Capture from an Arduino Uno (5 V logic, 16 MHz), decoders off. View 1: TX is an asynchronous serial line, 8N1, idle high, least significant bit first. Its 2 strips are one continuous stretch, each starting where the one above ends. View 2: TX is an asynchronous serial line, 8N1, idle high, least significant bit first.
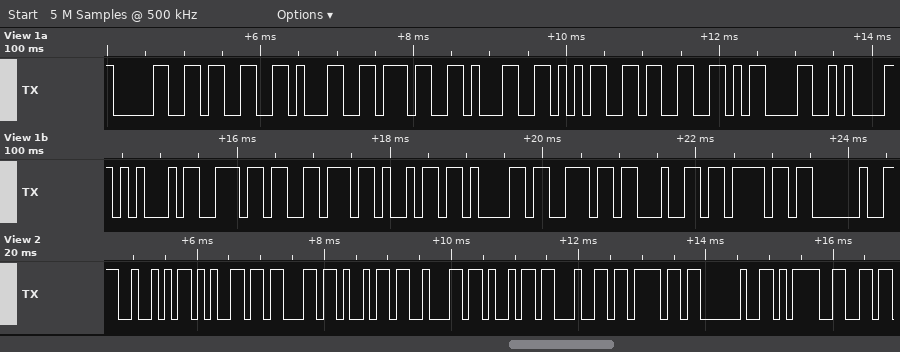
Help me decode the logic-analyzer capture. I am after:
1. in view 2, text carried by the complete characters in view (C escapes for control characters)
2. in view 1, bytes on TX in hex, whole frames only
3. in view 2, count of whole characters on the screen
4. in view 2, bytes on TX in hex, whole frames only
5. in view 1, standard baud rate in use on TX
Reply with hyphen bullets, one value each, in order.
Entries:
- "Recibido ="
- 0x30 0x33 0x31 0x37 0x31 0x35 0x33 0x0D 0x0A 0x45 0x6E 0x76 0x69 0x61 0x6E 0x64 0x6F 0x20
- 10
- 52 65 63 69 62 69 64 6F 20 3D
- 9600 baud
